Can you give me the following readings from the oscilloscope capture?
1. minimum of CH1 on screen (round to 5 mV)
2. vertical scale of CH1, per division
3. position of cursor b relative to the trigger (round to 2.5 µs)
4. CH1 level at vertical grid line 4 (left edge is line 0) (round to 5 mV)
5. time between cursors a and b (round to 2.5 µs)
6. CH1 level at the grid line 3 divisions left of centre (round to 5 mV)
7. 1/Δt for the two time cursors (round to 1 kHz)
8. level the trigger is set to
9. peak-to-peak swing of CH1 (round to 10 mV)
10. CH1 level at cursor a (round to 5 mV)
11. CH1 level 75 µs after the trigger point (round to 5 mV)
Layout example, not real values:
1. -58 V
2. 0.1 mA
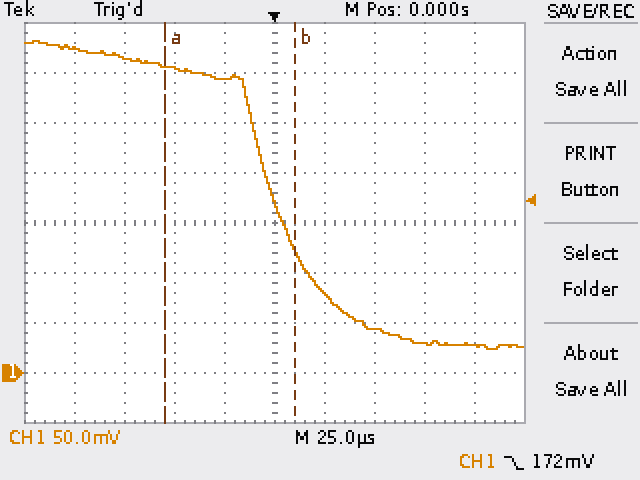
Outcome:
1. 25 mV
2. 50 mV
3. +10.0 µs
4. 295 mV
5. 65.0 µs
6. 315 mV
7. 15 kHz
8. 172 mV
9. 310 mV
10. 310 mV
11. 30 mV
